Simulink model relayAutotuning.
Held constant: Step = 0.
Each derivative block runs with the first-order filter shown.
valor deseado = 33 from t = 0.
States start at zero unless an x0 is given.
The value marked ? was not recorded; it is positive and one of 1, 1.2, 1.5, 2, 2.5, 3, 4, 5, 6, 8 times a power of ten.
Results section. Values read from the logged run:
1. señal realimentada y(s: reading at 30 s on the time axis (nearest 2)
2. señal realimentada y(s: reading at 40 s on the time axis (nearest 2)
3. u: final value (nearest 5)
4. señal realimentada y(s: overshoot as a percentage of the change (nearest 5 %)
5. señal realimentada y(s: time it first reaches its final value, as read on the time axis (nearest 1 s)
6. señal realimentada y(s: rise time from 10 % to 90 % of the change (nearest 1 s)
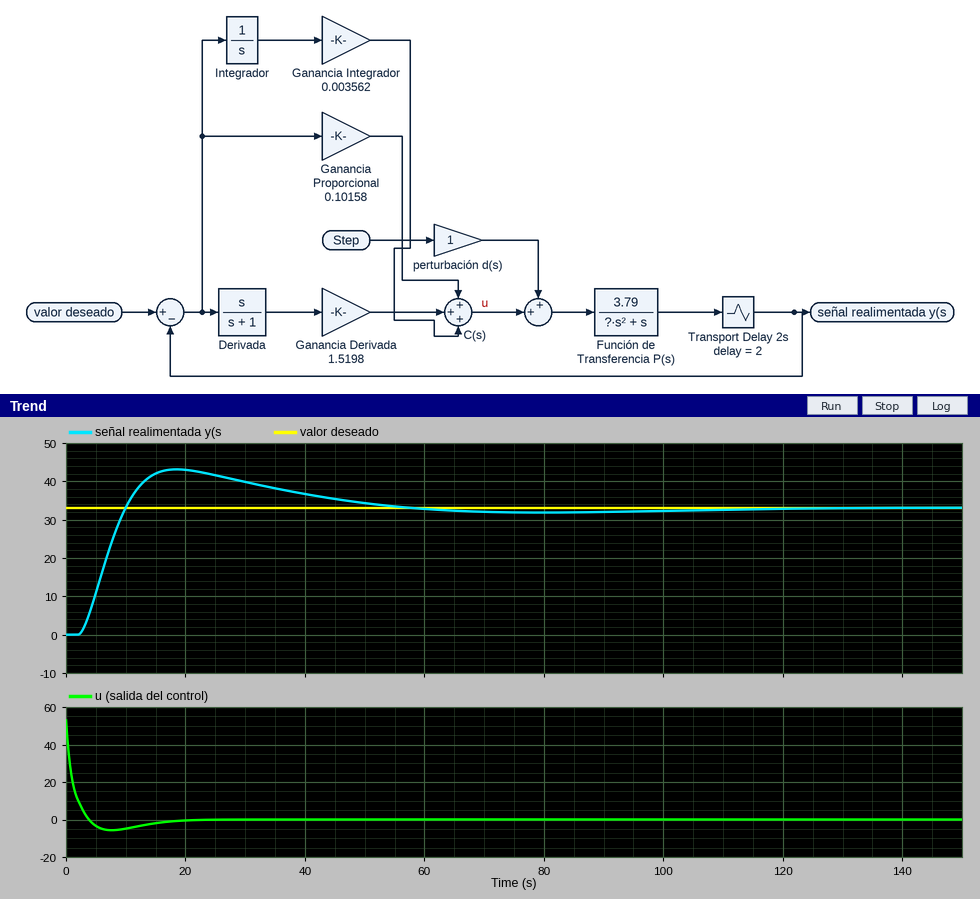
40
36
0
30 %
10 s
6 s
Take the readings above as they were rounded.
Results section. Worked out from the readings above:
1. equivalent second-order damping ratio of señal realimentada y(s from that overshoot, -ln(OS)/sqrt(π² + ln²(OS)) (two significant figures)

0.36
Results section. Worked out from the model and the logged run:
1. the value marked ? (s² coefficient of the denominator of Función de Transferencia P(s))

40
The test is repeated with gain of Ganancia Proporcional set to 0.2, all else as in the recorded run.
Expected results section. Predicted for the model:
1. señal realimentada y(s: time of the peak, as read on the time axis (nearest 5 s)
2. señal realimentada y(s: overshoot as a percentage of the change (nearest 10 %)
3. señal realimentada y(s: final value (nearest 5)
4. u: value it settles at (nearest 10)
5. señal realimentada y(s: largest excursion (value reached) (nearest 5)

15 s
50 %
35
0
50
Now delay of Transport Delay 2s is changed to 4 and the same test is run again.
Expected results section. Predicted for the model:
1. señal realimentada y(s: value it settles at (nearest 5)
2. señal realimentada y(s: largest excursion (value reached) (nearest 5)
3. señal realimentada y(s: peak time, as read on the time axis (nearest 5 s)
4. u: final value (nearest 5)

35
55
20 s
0
